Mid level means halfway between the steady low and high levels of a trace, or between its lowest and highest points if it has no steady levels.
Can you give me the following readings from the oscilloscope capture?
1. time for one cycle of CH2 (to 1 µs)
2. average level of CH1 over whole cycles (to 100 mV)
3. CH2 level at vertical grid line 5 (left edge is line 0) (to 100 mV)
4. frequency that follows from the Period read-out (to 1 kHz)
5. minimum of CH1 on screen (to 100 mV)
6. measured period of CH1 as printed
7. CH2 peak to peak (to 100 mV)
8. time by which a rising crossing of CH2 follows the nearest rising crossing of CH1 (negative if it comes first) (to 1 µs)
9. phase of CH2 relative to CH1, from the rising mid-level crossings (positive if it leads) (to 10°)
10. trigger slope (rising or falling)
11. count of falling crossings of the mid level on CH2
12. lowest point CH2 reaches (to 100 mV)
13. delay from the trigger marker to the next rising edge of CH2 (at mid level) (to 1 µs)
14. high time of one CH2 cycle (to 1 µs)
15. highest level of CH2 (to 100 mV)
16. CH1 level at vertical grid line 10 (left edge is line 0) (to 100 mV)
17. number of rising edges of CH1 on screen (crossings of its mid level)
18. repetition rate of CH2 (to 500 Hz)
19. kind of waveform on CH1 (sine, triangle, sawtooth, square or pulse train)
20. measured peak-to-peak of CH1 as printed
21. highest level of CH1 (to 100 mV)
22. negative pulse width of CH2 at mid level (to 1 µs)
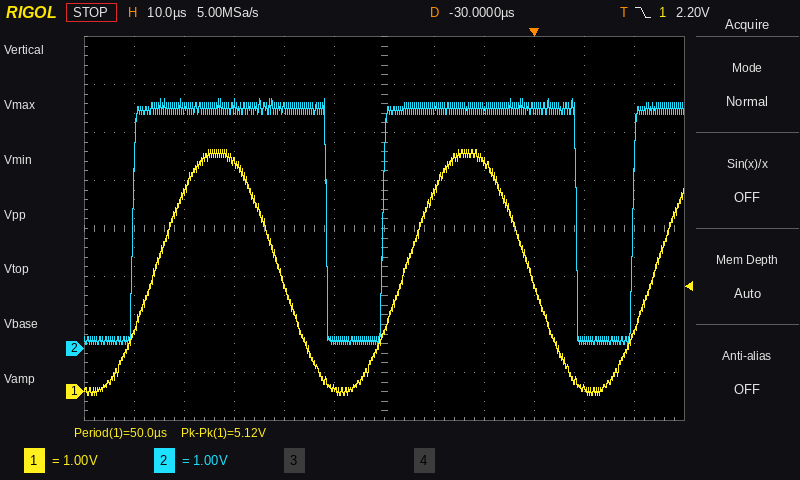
50 µs
2.5 V
200 mV
20 kHz
-100 mV
50.0 µs
5.1 V
-4 µs
+30°
falling
2
100 mV
20 µs
39 µs
5.2 V
100 mV
3
20.0 kHz
sine
5.12 V
5.0 V
11 µs
